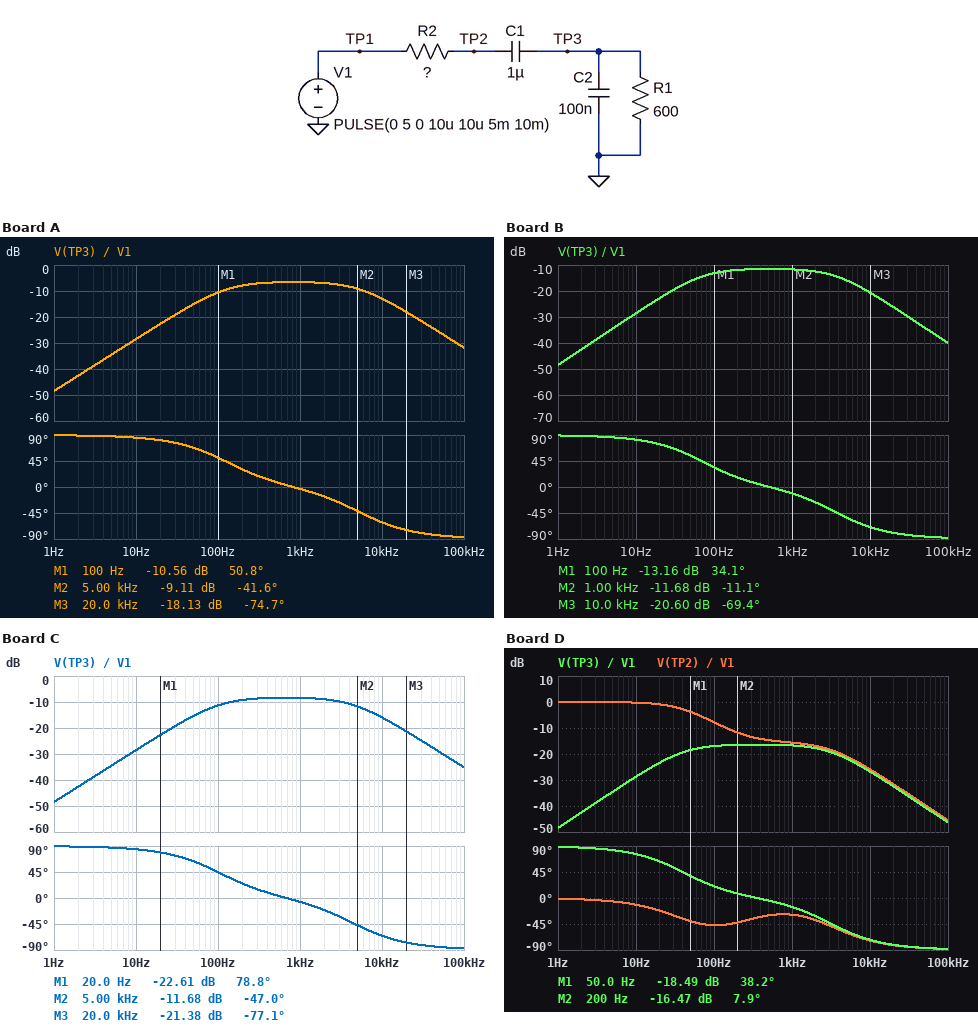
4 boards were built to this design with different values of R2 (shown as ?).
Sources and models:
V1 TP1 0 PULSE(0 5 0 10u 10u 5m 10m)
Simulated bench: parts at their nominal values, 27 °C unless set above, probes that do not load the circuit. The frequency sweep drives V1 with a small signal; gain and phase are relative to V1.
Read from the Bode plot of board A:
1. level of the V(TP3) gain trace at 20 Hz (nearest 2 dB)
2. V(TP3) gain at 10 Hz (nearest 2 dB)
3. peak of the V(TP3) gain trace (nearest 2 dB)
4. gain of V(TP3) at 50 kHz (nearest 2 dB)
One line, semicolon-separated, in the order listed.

-22 dB; -28 dB; -6 dB; -26 dB
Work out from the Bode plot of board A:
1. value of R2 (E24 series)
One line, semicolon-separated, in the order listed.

620 Ω
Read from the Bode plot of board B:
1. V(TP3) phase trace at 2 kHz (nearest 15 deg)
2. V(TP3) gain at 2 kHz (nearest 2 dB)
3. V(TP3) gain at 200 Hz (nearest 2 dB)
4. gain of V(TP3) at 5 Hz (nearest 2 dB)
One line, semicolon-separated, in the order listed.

-30 deg; -12 dB; -12 dB; -34 dB
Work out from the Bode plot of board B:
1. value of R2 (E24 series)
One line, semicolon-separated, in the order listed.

1.6 kΩ
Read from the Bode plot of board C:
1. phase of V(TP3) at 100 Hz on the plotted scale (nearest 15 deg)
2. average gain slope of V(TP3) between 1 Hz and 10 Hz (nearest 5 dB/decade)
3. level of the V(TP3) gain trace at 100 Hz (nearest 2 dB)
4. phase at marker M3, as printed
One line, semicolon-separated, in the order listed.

45 deg; 20 dB/decade; -12 dB; -77.1 deg
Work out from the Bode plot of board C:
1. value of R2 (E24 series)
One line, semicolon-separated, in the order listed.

910 Ω
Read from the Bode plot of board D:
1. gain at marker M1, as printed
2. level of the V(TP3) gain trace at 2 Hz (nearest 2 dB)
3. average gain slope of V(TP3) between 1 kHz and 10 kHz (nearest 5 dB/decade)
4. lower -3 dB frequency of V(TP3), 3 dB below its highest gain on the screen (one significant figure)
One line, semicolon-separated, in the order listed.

-18.49 dB; -42 dB; -10 dB/decade; 40 Hz
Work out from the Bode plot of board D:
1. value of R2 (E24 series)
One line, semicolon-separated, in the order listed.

3.3 kΩ
